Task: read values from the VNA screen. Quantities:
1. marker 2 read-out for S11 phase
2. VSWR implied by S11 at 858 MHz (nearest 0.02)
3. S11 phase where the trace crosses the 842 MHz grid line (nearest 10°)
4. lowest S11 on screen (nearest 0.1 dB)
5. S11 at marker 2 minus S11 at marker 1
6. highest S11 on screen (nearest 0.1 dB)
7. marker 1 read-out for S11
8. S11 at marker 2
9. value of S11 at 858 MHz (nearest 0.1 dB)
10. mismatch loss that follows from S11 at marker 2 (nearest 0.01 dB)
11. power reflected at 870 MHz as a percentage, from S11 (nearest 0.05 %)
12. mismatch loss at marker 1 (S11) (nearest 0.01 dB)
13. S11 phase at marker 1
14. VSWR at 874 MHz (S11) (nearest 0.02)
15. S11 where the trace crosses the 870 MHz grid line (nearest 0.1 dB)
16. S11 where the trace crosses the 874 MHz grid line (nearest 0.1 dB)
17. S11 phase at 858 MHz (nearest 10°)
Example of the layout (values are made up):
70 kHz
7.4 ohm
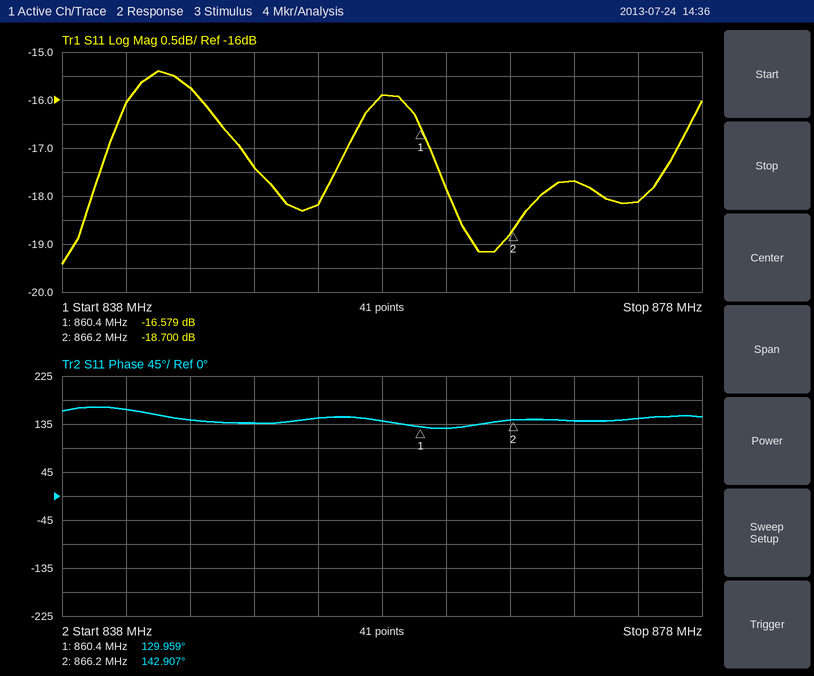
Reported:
142.907°
1.38
160°
-19.4 dB
-2.121 dB
-15.4 dB
-16.579 dB
-18.700 dB
-15.9 dB
0.06 dB
1.70 %
0.10 dB
129.959°
1.28
-17.7 dB
-18.1 dB
140°
